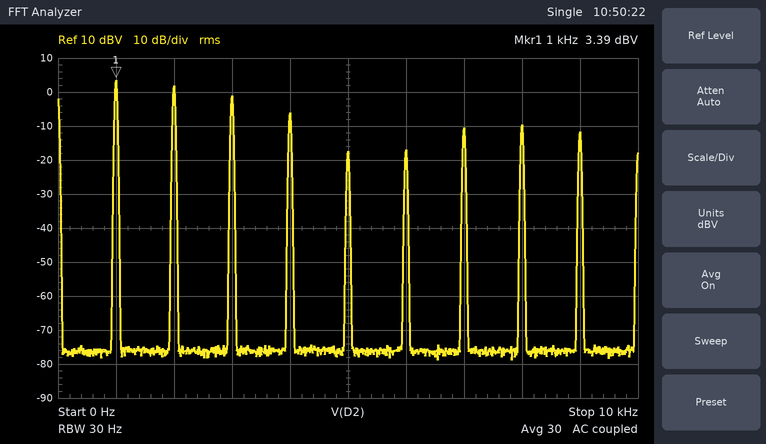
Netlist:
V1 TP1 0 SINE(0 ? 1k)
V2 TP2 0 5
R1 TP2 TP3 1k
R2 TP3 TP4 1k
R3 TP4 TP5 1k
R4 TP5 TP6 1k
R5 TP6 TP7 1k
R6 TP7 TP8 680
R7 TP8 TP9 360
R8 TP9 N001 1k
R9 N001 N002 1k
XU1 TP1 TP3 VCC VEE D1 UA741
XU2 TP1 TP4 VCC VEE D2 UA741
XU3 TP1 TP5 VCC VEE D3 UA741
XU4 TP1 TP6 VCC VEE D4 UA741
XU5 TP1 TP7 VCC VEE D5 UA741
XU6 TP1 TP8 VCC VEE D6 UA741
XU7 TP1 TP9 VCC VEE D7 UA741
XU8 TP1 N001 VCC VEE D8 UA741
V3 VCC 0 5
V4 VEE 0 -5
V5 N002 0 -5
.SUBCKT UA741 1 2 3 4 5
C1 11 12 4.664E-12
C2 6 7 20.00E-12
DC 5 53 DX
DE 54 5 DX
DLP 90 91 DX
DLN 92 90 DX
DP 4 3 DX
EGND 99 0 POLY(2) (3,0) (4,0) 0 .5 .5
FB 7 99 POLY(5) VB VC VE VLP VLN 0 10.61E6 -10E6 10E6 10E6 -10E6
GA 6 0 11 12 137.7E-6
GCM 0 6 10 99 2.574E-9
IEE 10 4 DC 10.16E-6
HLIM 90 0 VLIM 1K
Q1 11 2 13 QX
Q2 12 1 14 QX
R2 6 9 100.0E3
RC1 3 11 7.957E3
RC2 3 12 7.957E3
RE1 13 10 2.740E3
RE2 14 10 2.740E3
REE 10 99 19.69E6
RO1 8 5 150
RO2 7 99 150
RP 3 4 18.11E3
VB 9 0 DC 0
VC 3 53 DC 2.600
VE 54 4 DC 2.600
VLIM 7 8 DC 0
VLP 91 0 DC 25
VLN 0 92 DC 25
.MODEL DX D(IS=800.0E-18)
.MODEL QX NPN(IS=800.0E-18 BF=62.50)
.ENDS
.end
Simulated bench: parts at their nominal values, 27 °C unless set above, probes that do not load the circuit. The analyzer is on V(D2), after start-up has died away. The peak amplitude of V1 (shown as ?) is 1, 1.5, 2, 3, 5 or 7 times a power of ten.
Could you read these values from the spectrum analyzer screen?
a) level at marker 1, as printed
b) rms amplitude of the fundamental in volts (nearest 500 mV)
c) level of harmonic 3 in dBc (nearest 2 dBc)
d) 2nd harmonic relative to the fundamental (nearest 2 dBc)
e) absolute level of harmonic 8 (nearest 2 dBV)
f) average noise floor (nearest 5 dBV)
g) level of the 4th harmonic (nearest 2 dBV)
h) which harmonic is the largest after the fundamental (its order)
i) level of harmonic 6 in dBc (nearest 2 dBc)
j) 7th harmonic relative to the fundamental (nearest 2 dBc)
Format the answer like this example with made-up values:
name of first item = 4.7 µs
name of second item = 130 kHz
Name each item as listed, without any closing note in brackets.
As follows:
level at marker 1, as printed = 3.39 dBV
rms amplitude of the fundamental in volts = 1.5 V
level of harmonic 3 in dBc = -4 dBc
2nd harmonic relative to the fundamental = -2 dBc
absolute level of harmonic 8 = -10 dBV
average noise floor = -75 dBV
level of the 4th harmonic = -6 dBV
which harmonic is the largest after the fundamental = 2
level of harmonic 6 in dBc = -20 dBc
7th harmonic relative to the fundamental = -14 dBc
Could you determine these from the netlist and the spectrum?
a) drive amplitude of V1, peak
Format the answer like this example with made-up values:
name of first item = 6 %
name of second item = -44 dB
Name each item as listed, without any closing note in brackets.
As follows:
drive amplitude of V1, peak = 3 V
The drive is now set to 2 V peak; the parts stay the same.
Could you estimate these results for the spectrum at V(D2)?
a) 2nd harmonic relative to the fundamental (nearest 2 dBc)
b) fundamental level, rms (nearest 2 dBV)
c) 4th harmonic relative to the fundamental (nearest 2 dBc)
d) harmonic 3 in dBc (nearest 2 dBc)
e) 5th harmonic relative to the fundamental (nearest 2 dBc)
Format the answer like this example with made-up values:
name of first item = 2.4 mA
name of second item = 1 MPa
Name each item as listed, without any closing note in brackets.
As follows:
2nd harmonic relative to the fundamental = -20 dBc
fundamental level, rms = -152 dBV
4th harmonic relative to the fundamental = -28 dBc
harmonic 3 in dBc = -28 dBc
5th harmonic relative to the fundamental = -24 dBc
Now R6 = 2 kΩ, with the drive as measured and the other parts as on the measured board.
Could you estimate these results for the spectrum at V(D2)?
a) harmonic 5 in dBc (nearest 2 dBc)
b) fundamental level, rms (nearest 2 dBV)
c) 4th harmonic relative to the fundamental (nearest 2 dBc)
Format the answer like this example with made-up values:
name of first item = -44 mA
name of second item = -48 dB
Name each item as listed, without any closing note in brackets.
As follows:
harmonic 5 in dBc = -4 dBc
fundamental level, rms = -2 dBV
4th harmonic relative to the fundamental = -2 dBc
